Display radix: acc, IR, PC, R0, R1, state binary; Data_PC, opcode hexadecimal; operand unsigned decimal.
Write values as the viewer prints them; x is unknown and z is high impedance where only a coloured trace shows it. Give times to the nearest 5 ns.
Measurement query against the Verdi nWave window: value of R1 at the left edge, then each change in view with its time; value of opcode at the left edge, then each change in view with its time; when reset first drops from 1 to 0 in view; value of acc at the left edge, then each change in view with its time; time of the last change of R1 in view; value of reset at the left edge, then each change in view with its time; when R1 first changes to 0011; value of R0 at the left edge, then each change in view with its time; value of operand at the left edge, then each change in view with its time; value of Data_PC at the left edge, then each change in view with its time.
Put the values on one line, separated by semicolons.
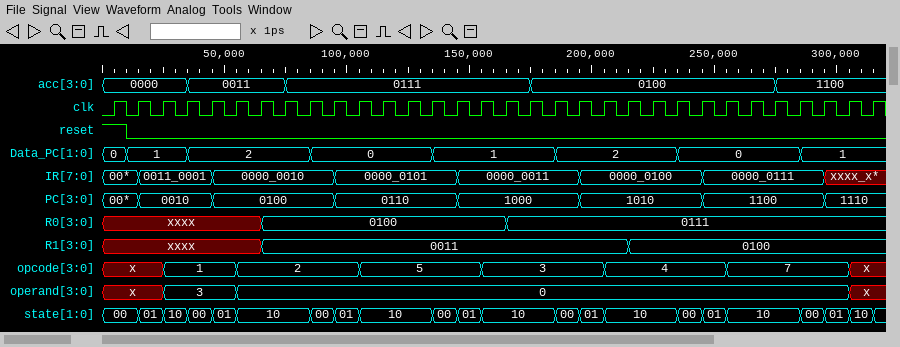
xxxx, 0011 at 65 ns, 0100 at 215 ns; x, 1 at 25 ns, 2 at 55 ns, 5 at 105 ns, 3 at 155 ns, 4 at 205 ns, 7 at 255 ns, x at 305 ns; 10 ns; 0000, 0011 at 35 ns, 0111 at 75 ns, 0100 at 175 ns, 1100 at 275 ns; 215 ns; 1, 0 at 10 ns; 65 ns; xxxx, 0100 at 65 ns, 0111 at 165 ns; x, 3 at 25 ns, 0 at 55 ns, x at 305 ns; 0, 1 at 10 ns, 2 at 35 ns, 0 at 85 ns, 1 at 135 ns, 2 at 185 ns, 0 at 235 ns, 1 at 285 ns
